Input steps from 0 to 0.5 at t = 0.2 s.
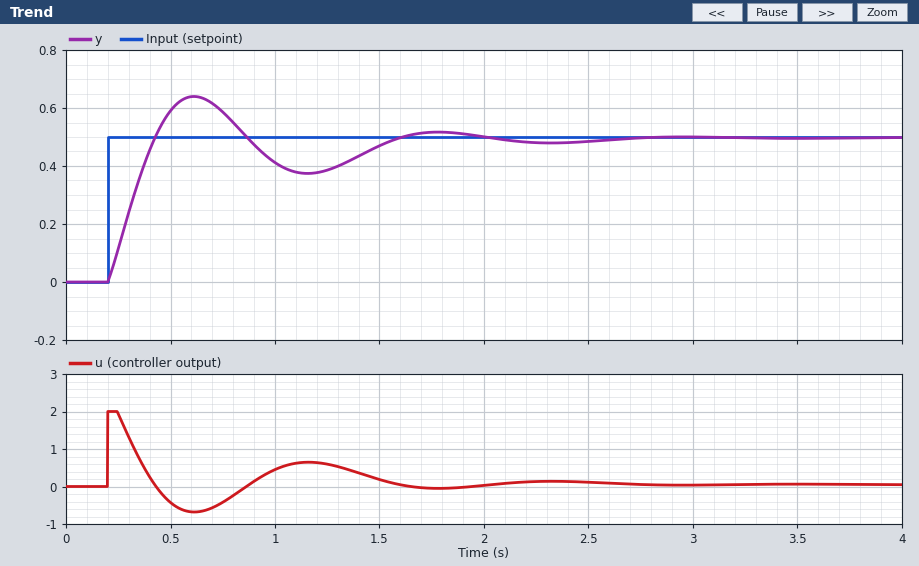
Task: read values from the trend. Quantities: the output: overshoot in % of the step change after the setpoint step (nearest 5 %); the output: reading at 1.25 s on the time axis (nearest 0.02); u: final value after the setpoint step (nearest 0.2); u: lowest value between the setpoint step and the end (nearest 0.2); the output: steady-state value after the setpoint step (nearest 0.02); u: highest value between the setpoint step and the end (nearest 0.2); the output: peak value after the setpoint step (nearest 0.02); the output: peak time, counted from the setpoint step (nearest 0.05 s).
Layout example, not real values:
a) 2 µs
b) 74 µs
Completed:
a) 30 %
b) 0.38
c) 0.0
d) -0.6
e) 0.50
f) 2.0
g) 0.64
h) 0.40 s
